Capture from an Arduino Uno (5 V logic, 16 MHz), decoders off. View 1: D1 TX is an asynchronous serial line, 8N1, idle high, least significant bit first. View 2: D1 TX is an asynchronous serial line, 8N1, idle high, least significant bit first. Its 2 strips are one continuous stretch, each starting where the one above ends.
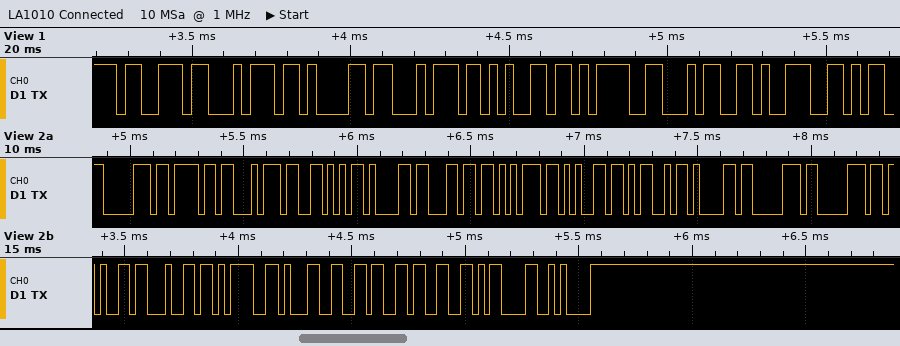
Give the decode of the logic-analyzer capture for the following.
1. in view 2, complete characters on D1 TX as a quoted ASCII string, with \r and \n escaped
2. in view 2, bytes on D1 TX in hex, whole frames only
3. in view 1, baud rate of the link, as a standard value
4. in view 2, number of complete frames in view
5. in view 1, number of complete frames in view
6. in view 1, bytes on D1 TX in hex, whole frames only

"potValueMapped=163\r\n"
70 6F 74 56 61 6C 75 65 4D 61 70 70 65 64 3D 31 36 33 0D 0A
38400 baud
20
8
73 74 61 74 65 3D 34 39
